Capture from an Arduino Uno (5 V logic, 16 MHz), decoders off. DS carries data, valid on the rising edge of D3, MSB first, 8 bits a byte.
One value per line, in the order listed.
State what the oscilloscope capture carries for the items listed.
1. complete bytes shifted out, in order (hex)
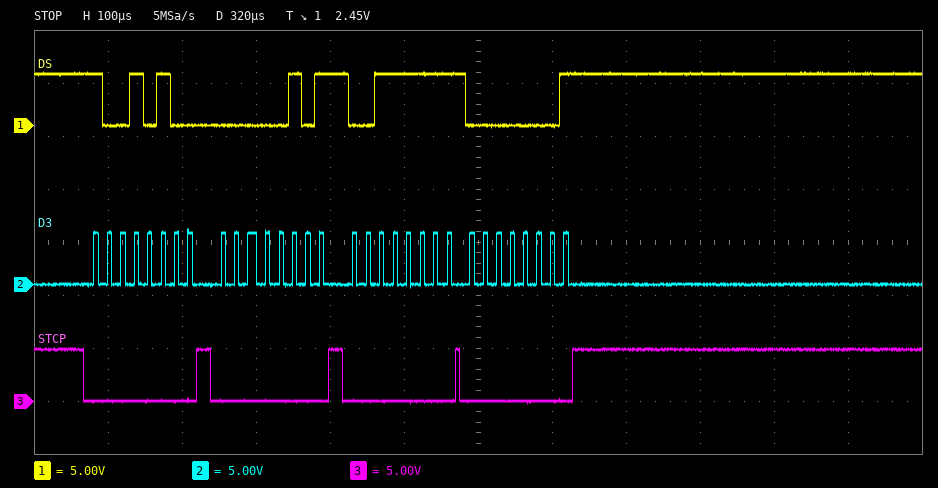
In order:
0x94 0x05 0x3F 0x01
